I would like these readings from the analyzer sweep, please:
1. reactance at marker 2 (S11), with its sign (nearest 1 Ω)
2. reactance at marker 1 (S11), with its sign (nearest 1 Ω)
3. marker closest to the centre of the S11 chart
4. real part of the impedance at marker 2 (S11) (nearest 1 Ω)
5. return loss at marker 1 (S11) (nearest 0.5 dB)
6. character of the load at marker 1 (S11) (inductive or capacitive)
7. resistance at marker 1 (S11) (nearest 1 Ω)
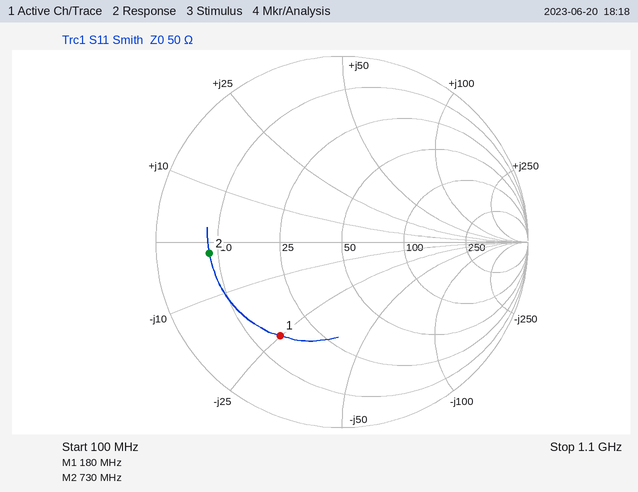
-2 Ω
-25 Ω
marker 1
8 Ω
4.5 dB
capacitive
16 Ω
